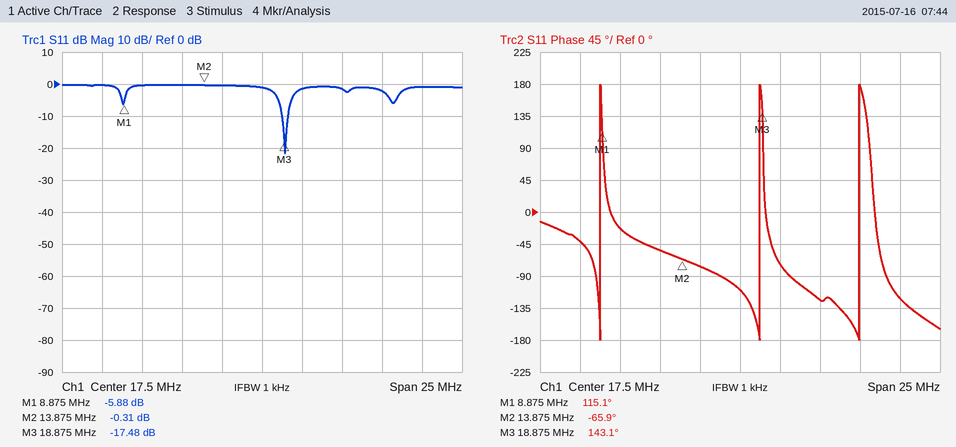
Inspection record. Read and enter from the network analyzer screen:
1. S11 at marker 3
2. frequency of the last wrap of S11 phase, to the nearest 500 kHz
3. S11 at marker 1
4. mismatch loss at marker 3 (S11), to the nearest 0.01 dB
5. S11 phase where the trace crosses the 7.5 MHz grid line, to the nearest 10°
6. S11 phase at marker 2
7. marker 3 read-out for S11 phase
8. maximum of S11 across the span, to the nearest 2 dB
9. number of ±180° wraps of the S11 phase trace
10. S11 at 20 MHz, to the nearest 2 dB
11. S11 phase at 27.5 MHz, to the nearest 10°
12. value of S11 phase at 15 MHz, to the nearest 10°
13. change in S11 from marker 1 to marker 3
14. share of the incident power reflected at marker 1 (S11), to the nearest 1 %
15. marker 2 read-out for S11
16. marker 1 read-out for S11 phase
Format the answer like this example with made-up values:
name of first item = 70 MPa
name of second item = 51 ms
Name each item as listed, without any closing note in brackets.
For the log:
S11 at marker 3 = -17.48 dB
frequency of the last wrap of S11 phase, to the nearest 500 kHz = 25.0 MHz
S11 at marker 1 = -5.88 dB
mismatch loss at marker 3 (S11), to the nearest 0.01 dB = 0.08 dB
S11 phase where the trace crosses the 7.5 MHz grid line, to the nearest 10° = -40°
S11 phase at marker 2 = -65.9°
marker 3 read-out for S11 phase = 143.1°
maximum of S11 across the span, to the nearest 2 dB = 0 dB
number of ±180° wraps of the S11 phase trace = 3
S11 at 20 MHz, to the nearest 2 dB = -2 dB
S11 phase at 27.5 MHz, to the nearest 10° = -120°
value of S11 phase at 15 MHz, to the nearest 10° = -80°
change in S11 from marker 1 to marker 3 = -11.60 dB
share of the incident power reflected at marker 1 (S11), to the nearest 1 % = 26 %
marker 2 read-out for S11 = -0.31 dB
marker 1 read-out for S11 phase = 115.1°
